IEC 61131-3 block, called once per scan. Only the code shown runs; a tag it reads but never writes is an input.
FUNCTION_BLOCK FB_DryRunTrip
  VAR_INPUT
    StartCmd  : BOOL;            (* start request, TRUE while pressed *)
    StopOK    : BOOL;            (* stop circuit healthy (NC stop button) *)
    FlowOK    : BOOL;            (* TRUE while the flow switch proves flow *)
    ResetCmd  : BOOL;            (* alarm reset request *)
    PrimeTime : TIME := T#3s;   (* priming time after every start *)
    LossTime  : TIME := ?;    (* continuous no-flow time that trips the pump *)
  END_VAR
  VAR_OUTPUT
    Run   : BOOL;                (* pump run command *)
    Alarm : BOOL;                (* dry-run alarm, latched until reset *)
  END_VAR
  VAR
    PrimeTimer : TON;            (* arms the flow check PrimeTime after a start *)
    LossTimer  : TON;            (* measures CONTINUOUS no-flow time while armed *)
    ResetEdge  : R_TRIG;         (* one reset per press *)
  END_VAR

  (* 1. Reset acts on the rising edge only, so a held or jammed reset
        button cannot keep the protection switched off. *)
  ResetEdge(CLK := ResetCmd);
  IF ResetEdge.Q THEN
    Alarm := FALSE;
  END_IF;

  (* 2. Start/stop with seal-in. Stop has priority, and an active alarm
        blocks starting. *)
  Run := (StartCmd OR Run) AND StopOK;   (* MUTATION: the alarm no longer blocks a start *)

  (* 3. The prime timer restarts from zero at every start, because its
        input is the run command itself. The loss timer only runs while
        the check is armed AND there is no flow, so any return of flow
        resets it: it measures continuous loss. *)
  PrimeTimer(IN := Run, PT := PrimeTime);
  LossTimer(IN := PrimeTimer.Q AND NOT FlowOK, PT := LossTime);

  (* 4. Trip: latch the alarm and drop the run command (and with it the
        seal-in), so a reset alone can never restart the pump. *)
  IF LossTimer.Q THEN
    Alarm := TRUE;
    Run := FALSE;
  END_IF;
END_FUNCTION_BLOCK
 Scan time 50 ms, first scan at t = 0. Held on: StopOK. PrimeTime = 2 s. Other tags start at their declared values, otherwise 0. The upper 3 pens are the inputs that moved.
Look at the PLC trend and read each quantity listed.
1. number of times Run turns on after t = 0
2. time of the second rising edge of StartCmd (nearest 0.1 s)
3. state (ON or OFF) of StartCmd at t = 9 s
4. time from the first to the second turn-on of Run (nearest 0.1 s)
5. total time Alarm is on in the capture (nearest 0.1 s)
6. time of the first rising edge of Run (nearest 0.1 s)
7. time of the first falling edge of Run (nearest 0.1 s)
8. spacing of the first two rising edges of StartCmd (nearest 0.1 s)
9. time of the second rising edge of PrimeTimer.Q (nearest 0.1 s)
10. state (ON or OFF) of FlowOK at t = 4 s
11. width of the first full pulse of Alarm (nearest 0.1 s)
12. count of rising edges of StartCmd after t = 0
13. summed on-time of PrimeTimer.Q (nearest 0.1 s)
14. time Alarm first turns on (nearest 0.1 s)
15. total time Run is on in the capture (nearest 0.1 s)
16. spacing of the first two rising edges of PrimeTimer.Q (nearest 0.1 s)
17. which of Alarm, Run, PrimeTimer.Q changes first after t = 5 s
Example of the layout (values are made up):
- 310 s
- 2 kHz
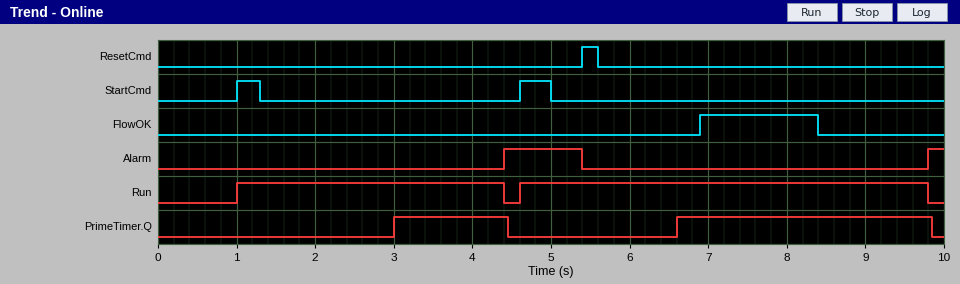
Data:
- 2
- 4.6 s
- OFF
- 3.6 s
- 1.2 s
- 1.0 s
- 4.4 s
- 3.6 s
- 6.6 s
- OFF
- 1.0 s
- 2
- 4.7 s
- 4.4 s
- 8.6 s
- 3.6 s
- Alarm
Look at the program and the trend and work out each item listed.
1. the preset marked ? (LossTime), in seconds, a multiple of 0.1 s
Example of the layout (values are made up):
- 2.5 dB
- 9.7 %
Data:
- 1.4 s
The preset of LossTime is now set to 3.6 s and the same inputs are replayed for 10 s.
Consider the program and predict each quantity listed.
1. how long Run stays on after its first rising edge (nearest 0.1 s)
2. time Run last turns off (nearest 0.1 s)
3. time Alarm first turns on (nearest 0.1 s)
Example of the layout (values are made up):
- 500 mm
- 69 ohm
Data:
- 5.6 s
- 6.6 s
- 6.6 s
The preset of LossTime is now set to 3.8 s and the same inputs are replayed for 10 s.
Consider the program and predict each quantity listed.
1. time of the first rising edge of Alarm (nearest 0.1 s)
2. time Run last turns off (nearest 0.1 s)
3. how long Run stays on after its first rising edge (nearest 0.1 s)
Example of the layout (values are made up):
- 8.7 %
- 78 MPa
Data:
- 6.8 s
- 6.8 s
- 5.8 s
